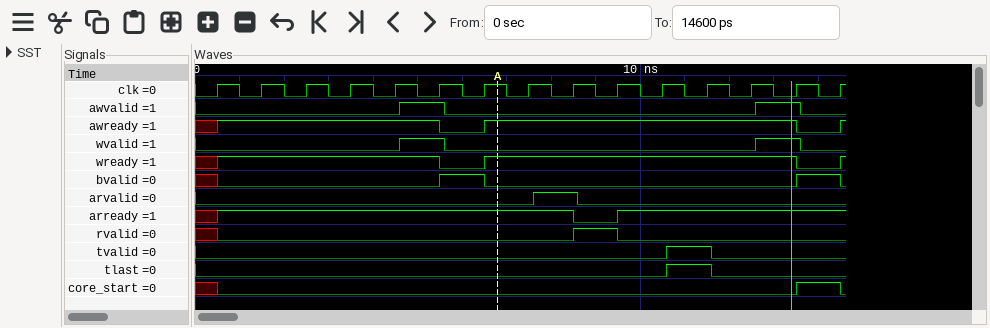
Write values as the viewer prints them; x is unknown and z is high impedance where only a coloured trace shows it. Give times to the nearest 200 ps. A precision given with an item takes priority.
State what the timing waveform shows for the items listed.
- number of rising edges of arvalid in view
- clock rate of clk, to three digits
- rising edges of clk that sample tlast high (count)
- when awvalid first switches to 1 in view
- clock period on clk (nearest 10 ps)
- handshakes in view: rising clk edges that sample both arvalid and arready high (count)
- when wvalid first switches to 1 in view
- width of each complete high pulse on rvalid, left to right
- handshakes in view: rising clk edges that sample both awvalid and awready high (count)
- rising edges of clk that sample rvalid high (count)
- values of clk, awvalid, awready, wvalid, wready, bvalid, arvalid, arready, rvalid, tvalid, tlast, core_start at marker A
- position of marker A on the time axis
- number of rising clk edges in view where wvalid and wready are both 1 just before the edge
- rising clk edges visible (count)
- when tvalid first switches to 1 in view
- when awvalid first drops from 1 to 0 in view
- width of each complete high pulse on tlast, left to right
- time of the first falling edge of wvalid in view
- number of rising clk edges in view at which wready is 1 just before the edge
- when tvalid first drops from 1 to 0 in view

1
1.00 GHz
1
4600 ps
1000 ps
1
4600 ps
1000 ps
2
1
clk=1, awvalid=0, awready=1, wvalid=0, wready=1, bvalid=0, arvalid=0, arready=1, rvalid=0, tvalid=0, tlast=0, core_start=0
6800 ps
2
15
10600 ps
5600 ps
1000 ps
5600 ps
12
11600 ps
